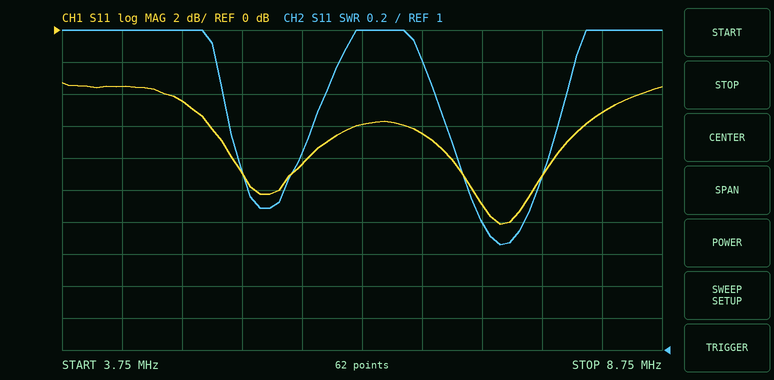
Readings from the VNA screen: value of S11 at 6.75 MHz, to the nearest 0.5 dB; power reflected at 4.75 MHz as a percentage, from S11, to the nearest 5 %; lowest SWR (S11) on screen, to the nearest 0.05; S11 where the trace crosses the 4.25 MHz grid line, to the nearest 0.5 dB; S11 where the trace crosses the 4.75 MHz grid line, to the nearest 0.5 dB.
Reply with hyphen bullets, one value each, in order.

- -6.5 dB
- 35 %
- 1.65
- -3.5 dB
- -4.5 dB
